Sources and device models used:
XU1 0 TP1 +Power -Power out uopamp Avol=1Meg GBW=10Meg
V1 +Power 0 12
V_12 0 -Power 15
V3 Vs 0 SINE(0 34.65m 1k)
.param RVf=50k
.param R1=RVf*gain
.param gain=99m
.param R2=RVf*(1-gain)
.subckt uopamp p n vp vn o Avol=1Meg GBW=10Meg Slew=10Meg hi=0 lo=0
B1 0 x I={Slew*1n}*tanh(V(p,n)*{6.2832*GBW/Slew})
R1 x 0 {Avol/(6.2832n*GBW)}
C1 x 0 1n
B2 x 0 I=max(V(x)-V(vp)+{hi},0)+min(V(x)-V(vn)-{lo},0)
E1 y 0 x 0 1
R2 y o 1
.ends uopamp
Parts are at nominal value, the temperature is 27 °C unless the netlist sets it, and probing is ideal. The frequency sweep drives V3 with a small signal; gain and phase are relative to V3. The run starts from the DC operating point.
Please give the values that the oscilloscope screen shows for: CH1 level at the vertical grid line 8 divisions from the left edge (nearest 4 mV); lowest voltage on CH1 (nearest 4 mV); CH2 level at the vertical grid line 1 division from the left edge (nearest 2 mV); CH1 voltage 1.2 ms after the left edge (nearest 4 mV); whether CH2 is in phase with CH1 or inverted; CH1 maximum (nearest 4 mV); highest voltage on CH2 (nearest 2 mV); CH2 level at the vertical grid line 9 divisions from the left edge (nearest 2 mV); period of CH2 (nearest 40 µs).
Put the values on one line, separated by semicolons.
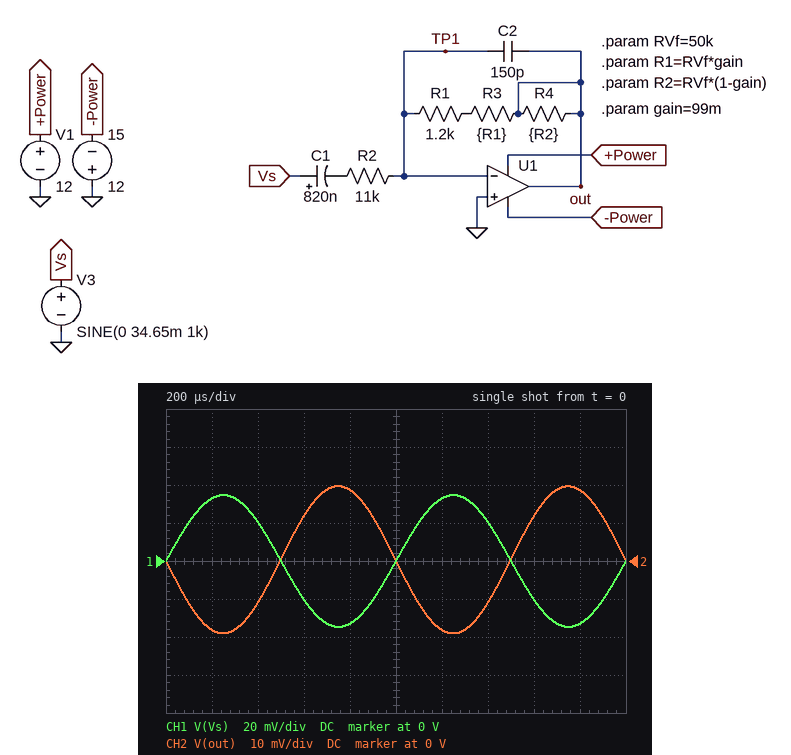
-20 mV; -36 mV; -18 mV; 32 mV; inverted; 36 mV; 20 mV; 18 mV; 1.00 ms
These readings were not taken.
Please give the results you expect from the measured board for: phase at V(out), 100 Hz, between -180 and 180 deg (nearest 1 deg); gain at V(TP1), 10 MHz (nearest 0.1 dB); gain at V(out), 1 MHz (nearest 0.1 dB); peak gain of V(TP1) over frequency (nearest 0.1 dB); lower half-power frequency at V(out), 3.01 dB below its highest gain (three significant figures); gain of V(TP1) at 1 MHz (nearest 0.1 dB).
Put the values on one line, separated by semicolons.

-170 deg; -43.4 dB; -20.6 dB; -40.5 dB; 17.6 Hz; -40.6 dB
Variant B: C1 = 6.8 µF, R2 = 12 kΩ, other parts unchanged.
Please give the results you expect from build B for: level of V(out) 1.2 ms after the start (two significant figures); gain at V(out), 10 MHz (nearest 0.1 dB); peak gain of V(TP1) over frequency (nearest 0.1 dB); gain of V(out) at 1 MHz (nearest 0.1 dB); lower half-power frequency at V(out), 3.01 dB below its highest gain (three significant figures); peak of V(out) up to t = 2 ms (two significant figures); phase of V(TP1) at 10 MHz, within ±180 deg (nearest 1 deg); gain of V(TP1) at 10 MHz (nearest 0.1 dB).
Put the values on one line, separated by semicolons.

-17 mV; -44.0 dB; -41.3 dB; -21.3 dB; 1.95 Hz; 18 mV; -43 deg; -44.1 dB
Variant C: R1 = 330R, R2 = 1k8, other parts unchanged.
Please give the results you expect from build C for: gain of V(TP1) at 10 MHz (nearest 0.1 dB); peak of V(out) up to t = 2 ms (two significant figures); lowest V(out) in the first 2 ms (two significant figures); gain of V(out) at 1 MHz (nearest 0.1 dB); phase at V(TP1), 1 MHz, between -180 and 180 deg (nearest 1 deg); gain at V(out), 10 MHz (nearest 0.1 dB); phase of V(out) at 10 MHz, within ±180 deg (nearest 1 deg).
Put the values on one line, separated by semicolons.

-27.9 dB; 110 mV; -96 mV; -5.3 dB; 5 deg; -27.8 dB; 48 deg
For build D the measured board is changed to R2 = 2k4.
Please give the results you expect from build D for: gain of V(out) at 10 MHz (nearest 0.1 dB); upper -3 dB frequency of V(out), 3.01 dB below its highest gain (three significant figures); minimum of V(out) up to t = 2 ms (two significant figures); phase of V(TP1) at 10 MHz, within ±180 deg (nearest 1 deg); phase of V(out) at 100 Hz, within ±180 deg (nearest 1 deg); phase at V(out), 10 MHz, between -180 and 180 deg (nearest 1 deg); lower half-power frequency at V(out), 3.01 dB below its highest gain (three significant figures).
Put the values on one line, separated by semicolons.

-30.2 dB; 165 kHz; -85 mV; -42 deg; -141 deg; 47 deg; 80.8 Hz
